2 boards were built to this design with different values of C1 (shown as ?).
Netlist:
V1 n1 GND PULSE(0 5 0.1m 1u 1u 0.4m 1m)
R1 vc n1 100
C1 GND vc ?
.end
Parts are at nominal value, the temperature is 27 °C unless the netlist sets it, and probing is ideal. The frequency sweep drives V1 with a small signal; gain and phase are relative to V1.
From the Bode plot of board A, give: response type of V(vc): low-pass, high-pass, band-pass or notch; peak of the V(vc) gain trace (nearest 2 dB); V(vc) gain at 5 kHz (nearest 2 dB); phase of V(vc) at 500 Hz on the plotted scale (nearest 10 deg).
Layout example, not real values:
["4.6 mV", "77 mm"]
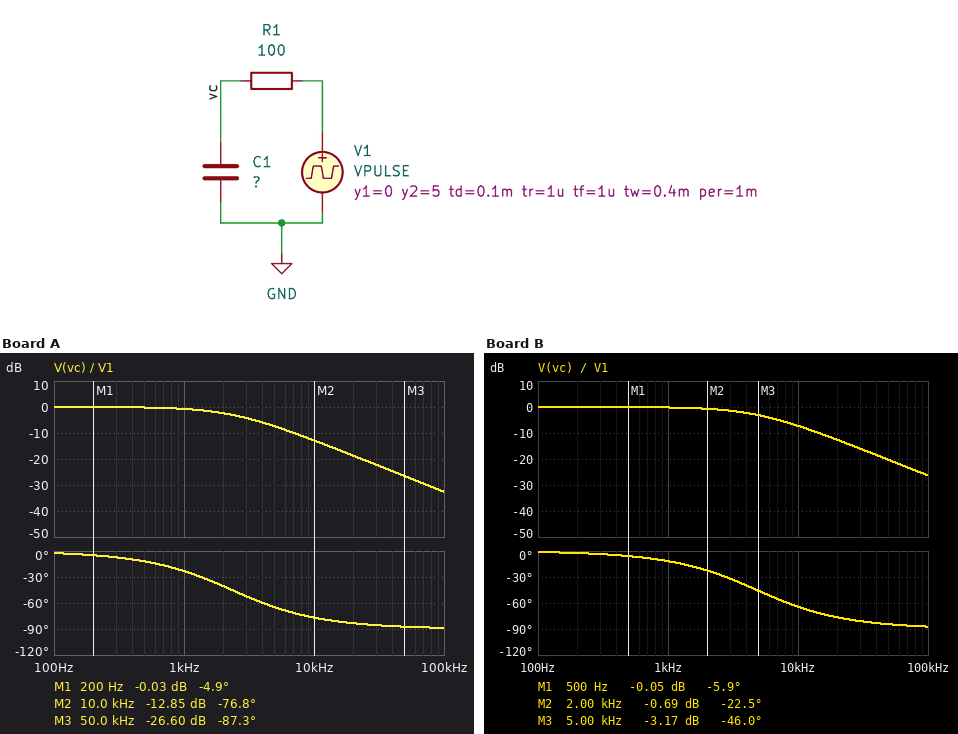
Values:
["low-pass", "0 dB", "-8 dB", "-10 deg"]
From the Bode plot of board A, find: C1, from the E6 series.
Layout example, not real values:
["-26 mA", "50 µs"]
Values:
["680 nF"]
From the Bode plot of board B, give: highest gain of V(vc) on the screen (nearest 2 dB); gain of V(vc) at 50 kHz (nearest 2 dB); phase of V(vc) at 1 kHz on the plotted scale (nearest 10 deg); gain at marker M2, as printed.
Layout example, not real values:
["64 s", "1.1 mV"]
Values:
["0 dB", "-20 dB", "-10 deg", "-0.69 dB"]
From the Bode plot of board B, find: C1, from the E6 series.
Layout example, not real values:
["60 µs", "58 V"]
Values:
["330 nF"]
